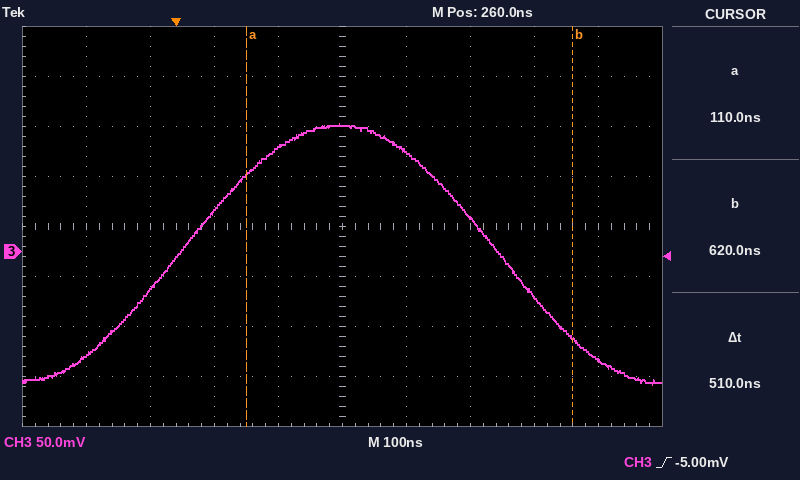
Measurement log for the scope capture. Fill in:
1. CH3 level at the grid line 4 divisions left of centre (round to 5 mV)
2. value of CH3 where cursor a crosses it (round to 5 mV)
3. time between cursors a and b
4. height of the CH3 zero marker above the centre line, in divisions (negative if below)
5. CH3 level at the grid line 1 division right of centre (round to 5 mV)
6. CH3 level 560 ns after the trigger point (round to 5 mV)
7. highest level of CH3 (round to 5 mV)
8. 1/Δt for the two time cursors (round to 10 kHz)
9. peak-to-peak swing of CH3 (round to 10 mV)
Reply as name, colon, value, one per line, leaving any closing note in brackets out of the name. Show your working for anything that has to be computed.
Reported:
CH3 level at the grid line 4 divisions left of centre: -105 mV
value of CH3 where cursor a crosses it: 80 mV
time between cursors a and b: 510 ns
height of the CH3 zero marker above the centre line, in divisions: -0.5 div
CH3 level at the grid line 1 division right of centre: 100 mV
CH3 level 560 ns after the trigger point: -45 mV
highest level of CH3: 130 mV
1/Δt for the two time cursors: 1 / 510 ns ≈ 1.96 MHz
peak-to-peak swing of CH3: 260 mV
